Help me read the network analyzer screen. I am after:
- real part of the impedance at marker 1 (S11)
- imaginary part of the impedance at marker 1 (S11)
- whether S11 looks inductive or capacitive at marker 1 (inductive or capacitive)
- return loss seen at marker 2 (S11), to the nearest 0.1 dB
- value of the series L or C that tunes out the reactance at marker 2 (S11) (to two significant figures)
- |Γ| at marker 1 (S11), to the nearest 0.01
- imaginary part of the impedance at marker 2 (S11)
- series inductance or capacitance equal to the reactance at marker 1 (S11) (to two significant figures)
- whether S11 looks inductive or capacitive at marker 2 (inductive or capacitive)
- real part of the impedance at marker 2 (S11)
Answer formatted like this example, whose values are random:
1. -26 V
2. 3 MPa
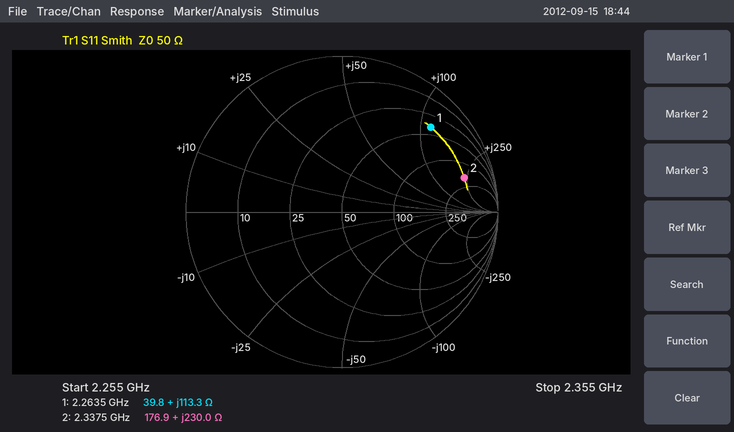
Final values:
1. 39.8 Ω
2. +113.3 Ω
3. inductive
4. 1.8 dB
5. 300 fF
6. 0.79
7. +230.0 Ω
8. 8.0 nH
9. inductive
10. 176.9 Ω
